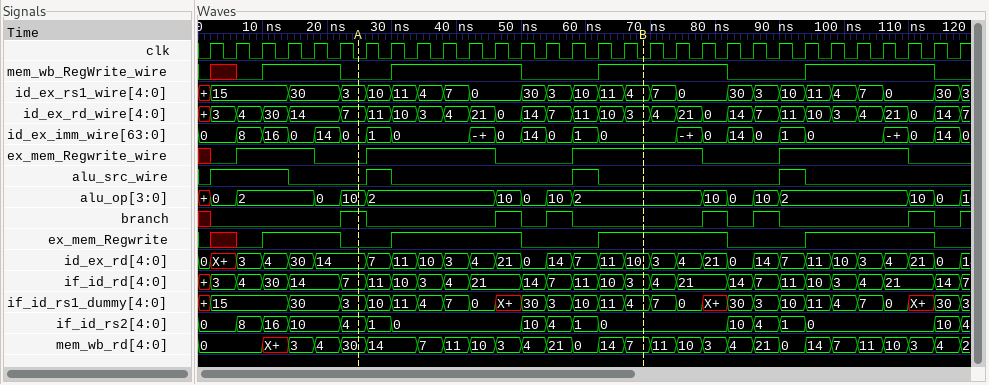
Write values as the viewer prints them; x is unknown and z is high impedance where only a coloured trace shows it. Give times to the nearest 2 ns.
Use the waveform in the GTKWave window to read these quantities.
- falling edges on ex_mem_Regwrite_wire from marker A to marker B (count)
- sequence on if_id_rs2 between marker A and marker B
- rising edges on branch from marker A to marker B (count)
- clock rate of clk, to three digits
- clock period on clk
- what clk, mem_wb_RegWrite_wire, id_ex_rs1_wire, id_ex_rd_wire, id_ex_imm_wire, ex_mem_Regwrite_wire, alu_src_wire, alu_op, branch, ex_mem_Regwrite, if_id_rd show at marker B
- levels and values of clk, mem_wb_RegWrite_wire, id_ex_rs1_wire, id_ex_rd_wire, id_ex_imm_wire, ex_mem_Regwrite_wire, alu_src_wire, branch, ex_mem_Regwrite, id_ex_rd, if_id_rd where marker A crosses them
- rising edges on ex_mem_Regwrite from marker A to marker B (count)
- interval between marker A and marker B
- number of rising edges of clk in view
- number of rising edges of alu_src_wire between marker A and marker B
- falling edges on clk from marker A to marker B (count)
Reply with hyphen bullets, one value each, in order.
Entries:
- 1
- 4, 1, 0, 10, 4, 1, 0
- 2
- 250 MHz
- 4 ns
- clk=0, mem_wb_RegWrite_wire=1, id_ex_rs1_wire=4, id_ex_rd_wire=3, id_ex_imm_wire=0, ex_mem_Regwrite_wire=1, alu_src_wire=0, alu_op=2, branch=0, ex_mem_Regwrite=1, if_id_rd=3
- clk=0, mem_wb_RegWrite_wire=0, id_ex_rs1_wire=3, id_ex_rd_wire=7, id_ex_imm_wire=0, ex_mem_Regwrite_wire=0, alu_src_wire=0, branch=1, ex_mem_Regwrite=0, id_ex_rd=14, if_id_rd=7
- 2
- 44 ns
- 30
- 2
- 11
